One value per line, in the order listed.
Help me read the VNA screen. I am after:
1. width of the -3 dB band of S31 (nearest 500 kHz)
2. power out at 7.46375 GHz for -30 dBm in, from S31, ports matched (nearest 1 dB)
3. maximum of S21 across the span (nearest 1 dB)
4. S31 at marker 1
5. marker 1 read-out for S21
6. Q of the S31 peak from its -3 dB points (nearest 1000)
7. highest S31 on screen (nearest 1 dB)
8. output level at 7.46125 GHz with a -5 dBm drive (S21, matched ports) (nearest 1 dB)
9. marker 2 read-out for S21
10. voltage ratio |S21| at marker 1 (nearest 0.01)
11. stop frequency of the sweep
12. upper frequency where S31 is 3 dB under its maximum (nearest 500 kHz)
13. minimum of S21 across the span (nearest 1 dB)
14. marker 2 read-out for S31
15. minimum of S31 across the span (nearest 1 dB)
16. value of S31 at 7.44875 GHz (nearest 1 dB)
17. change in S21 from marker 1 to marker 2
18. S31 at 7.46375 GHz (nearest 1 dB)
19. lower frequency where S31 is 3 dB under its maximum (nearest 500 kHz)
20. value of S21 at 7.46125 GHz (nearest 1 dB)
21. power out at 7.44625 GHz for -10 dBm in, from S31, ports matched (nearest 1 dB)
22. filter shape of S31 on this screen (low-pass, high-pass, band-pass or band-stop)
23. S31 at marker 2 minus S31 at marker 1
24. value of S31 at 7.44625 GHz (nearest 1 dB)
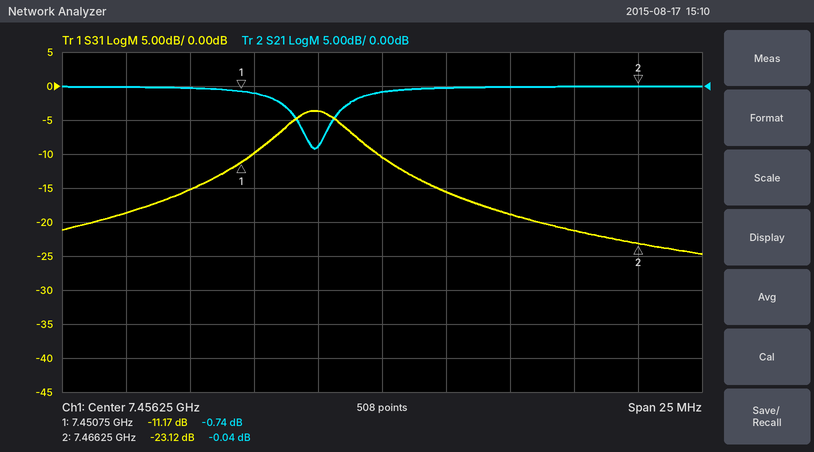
2.5 MHz
-51 dBm
0 dB
-11.17 dB
-0.74 dB
3000
-4 dB
-5 dBm
-0.04 dB
0.92
7.46875 GHz
7.4550 GHz
-9 dB
-23.12 dB
-25 dB
-15 dB
0.70 dB
-21 dB
7.4525 GHz
0 dB
-29 dBm
band-pass
-11.95 dB
-19 dB
